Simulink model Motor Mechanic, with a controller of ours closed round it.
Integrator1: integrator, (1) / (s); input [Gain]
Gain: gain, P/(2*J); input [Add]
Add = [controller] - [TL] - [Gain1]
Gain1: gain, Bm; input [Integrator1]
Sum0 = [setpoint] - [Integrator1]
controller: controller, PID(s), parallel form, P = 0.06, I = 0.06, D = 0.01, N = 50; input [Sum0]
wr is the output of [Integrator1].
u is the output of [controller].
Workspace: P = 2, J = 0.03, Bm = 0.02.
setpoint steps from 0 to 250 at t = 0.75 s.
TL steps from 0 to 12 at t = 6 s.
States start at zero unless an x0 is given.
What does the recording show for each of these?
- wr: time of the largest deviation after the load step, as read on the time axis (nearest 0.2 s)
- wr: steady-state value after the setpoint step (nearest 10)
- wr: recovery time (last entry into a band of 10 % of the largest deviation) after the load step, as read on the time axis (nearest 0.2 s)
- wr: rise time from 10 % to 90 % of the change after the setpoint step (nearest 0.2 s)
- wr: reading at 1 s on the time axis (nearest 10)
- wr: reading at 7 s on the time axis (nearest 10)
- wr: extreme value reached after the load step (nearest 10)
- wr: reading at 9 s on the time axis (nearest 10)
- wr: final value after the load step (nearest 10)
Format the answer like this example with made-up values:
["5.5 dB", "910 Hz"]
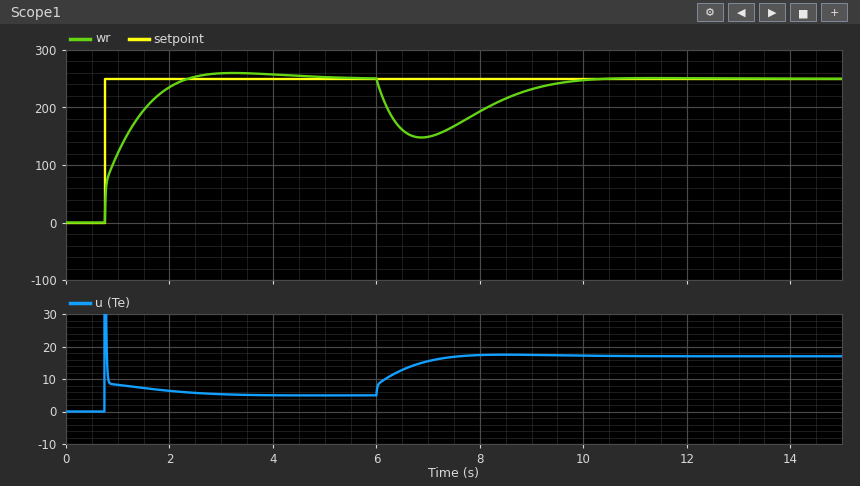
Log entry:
["6.8 s", "250", "9.4 s", "1.0 s", "120", "150", "150", "230", "250"]
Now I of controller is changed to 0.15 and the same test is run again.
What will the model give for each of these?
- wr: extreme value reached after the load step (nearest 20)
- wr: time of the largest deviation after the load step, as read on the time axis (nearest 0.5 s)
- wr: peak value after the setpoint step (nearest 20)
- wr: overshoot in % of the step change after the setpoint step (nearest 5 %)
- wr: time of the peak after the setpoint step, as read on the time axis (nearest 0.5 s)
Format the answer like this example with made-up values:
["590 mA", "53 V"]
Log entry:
["160", "6.5 s", "280", "15 %", "2.0 s"]
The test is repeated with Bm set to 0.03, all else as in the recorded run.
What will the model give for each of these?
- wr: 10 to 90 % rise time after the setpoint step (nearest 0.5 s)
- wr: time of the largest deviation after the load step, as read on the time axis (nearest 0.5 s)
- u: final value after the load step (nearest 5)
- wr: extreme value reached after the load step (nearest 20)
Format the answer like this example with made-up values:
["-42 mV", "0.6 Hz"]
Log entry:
["1.5 s", "7.0 s", "20", "160"]
